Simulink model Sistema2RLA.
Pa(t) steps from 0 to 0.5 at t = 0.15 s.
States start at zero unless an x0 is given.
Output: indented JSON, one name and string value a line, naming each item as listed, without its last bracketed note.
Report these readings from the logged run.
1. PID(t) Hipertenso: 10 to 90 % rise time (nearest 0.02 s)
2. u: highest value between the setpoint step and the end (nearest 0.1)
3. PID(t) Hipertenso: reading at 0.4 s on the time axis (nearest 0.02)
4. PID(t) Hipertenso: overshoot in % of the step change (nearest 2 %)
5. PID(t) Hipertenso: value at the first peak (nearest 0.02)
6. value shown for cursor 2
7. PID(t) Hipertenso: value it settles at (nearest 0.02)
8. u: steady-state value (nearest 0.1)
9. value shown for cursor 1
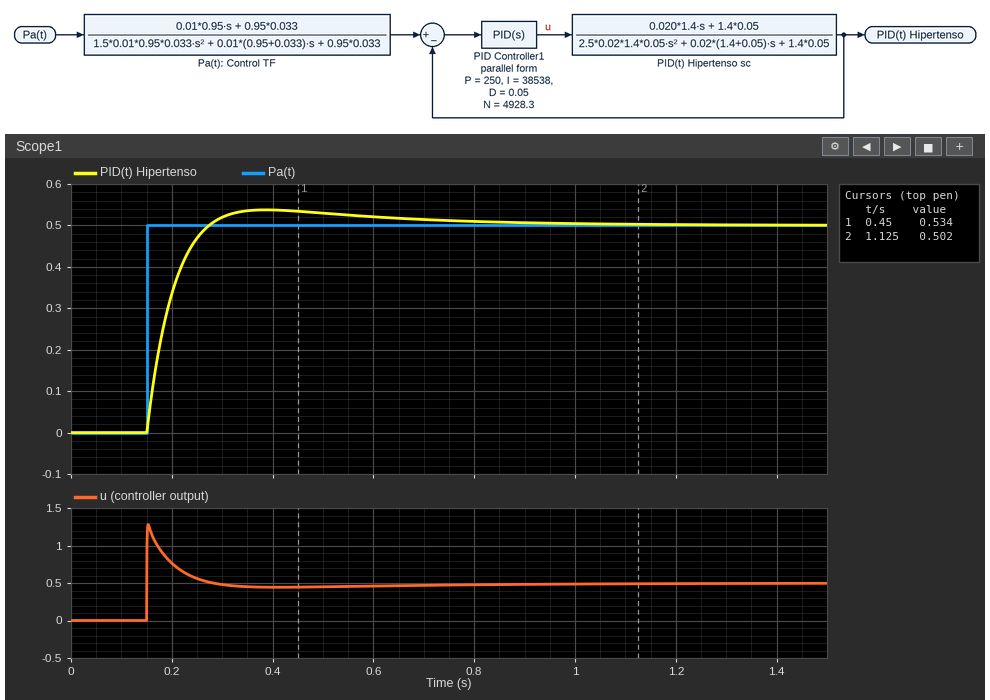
{
  "PID(t) Hipertenso: 10 to 90 % rise time": "0.08 s",
  "u: highest value between the setpoint step and the end": "1.3",
  "PID(t) Hipertenso: reading at 0.4 s on the time axis": "0.54",
  "PID(t) Hipertenso: overshoot in % of the step change": "8 %",
  "PID(t) Hipertenso: value at the first peak": "0.54",
  "value shown for cursor 2": "0.502",
  "PID(t) Hipertenso: value it settles at": "0.50",
  "u: steady-state value": "0.5",
  "value shown for cursor 1": "0.534"
}
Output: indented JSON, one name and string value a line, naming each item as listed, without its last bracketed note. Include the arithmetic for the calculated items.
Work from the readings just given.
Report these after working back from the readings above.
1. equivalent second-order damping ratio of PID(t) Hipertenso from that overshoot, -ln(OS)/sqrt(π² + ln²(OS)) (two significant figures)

{
  "equivalent second-order damping ratio of PID(t) Hipertenso from that overshoot, -ln(OS)/sqrt(π² + ln²(OS))": "ln(0.08) = -2.526; 2.526 / sqrt(9.870 + 6.379) = 0.63"
}
